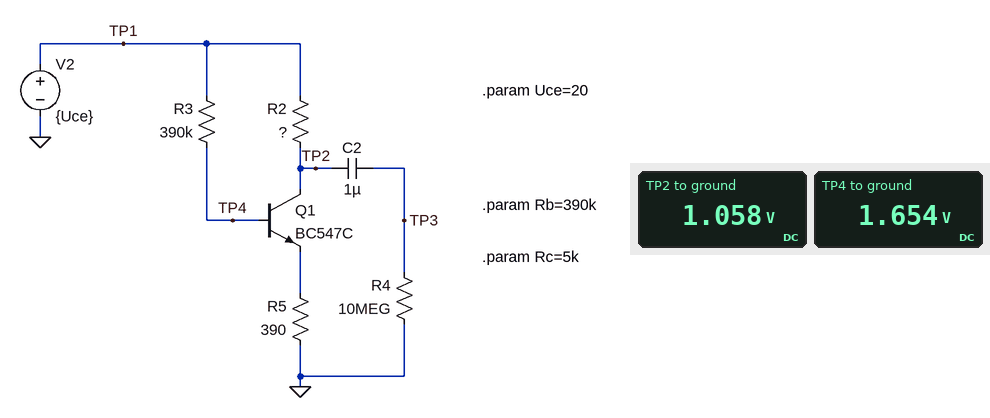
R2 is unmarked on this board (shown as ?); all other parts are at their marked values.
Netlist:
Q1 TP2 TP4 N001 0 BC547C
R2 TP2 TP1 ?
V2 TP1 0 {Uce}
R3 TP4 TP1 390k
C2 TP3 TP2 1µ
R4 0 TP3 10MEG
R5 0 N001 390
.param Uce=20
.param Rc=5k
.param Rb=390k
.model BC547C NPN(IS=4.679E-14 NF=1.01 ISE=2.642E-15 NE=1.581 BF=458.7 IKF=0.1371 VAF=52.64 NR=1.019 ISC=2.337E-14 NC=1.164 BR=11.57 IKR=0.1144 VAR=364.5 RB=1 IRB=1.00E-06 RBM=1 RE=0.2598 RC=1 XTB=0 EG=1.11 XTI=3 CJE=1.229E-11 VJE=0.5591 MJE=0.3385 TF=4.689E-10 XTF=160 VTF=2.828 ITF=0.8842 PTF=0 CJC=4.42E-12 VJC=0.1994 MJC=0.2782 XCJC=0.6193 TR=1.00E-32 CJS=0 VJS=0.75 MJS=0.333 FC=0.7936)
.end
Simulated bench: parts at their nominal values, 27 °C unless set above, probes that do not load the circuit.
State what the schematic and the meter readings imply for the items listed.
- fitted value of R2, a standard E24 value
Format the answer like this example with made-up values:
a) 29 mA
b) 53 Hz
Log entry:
a) 7.5 kΩ
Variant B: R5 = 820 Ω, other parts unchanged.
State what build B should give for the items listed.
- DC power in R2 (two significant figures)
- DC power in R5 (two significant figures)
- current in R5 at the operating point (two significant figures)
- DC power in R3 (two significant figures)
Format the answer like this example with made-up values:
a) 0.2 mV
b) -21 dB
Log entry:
a) 43 mW
b) 4.9 mW
c) 2.4 mA
d) 770 µW
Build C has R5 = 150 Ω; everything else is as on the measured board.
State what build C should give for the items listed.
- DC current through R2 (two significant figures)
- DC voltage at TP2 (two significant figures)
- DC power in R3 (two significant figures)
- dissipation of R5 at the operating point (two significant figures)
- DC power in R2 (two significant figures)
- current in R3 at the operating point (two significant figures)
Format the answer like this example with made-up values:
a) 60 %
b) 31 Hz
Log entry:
a) 2.6 mA
b) 450 mV
c) 920 µW
d) 1.1 mW
e) 51 mW
f) 49 µA
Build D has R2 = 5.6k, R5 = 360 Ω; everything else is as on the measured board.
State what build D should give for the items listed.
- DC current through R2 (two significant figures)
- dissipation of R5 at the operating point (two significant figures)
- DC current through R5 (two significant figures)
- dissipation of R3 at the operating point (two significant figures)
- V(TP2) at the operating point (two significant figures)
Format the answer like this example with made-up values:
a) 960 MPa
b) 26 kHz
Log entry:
a) 3.3 mA
b) 4.1 mW
c) 3.4 mA
d) 840 µW
e) 1.3 V
